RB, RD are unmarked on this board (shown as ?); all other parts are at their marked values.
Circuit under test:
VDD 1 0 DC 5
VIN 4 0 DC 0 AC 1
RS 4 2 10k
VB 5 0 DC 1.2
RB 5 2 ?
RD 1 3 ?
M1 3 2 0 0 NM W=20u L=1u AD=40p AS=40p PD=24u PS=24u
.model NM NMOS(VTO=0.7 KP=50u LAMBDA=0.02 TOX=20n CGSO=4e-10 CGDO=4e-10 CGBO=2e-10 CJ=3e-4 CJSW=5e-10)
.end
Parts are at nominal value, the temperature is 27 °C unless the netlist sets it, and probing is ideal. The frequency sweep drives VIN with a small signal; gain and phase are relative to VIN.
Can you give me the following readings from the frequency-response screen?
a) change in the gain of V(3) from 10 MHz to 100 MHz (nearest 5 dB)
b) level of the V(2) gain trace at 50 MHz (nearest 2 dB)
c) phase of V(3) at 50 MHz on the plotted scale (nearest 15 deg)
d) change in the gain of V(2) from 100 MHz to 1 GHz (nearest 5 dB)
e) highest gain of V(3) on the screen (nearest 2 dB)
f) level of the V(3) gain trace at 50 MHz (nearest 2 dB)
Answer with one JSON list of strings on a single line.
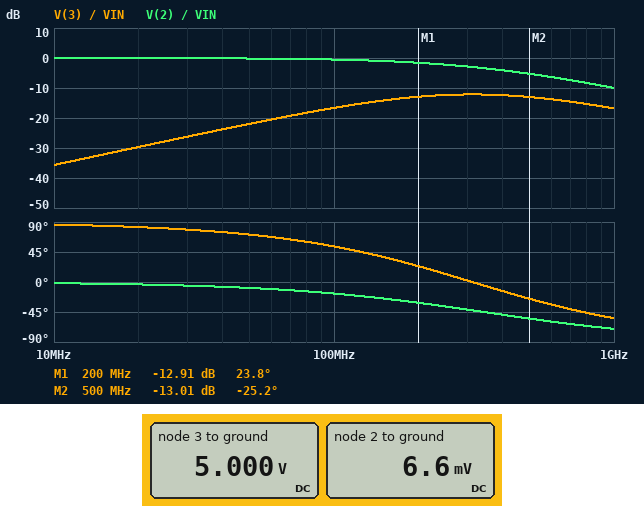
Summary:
["20 dB", "0 dB", "75 deg", "-10 dB", "-12 dB", "-22 dB"]
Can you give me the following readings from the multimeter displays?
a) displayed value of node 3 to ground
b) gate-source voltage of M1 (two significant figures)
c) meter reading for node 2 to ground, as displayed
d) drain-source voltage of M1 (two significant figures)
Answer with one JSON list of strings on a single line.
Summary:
["5.000 V", "6.6 mV", "6.6 mV", "5.0 V"]
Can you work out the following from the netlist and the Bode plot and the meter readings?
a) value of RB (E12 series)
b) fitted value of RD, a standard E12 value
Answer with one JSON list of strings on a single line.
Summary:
["1.8 MΩ", "33 kΩ"]
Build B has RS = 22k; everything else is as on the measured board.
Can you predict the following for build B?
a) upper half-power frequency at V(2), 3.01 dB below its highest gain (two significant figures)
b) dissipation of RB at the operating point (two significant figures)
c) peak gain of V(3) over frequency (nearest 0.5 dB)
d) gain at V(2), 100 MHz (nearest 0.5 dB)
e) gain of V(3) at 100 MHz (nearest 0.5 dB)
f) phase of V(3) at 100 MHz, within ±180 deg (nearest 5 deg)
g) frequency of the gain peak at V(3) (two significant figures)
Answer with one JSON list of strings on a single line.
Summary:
["140 MHz", "780 nW", "-16.0 dB", "-2.0 dB", "-18.0 dB", "35 deg", "210 MHz"]
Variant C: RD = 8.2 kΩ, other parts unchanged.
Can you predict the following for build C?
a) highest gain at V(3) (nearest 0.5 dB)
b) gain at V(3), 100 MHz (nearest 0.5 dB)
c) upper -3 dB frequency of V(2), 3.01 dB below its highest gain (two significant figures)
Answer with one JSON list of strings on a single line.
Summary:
["-20.0 dB", "-28.0 dB", "310 MHz"]
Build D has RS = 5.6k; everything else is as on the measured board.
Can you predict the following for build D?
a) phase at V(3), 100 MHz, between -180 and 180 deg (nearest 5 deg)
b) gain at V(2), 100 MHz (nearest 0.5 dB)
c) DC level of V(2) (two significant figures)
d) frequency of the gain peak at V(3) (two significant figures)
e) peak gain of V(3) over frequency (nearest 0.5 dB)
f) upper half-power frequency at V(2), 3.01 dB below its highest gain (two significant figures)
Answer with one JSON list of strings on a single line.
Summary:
["60 deg", "0 dB", "3.7 mV", "420 MHz", "-10.0 dB", "580 MHz"]
